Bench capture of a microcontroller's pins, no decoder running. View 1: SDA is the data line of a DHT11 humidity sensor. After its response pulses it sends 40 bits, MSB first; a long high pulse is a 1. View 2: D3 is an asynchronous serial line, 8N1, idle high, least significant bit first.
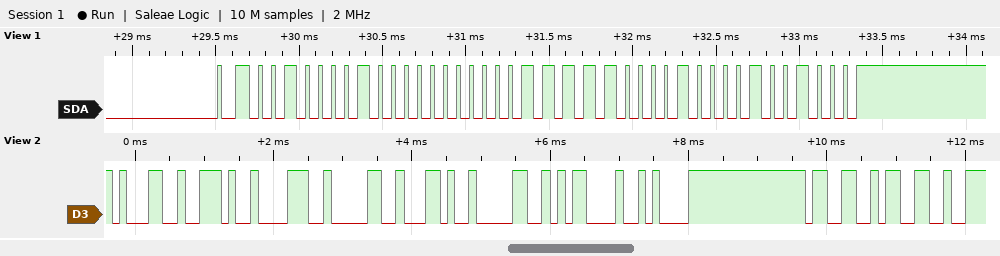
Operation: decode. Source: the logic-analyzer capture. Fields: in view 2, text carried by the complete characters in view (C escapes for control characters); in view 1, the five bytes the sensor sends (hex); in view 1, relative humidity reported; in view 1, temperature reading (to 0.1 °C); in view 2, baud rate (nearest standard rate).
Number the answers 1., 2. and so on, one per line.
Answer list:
1. "1.80,0\r\n33"
2. 21 00 1F 08 48
3. 33 %
4. 31.8 °C
5. 9600 baud
